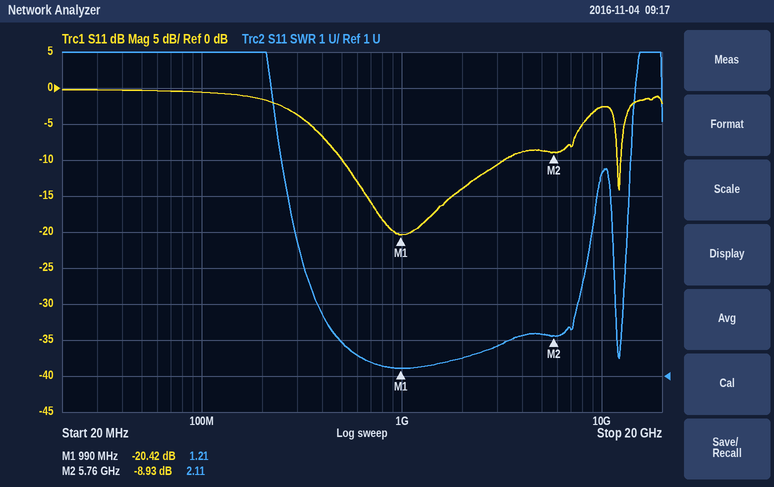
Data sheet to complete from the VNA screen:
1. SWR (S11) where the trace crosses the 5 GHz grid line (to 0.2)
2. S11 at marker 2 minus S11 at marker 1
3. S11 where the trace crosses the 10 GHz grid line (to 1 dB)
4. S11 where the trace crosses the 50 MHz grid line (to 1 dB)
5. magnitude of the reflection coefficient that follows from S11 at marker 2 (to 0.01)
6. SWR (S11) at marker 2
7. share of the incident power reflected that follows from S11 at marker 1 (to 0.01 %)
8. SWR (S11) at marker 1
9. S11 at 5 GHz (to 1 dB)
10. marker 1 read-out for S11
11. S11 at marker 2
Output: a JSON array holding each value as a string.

["2.2", "11.49 dB", "-3 dB", "0 dB", "0.36", "2.11", "0.91 %", "1.21", "-9 dB", "-20.42 dB", "-8.93 dB"]
